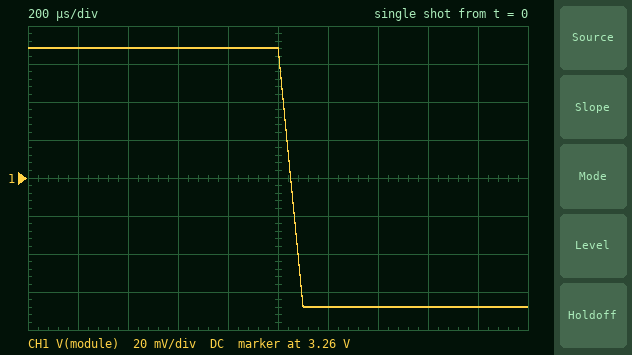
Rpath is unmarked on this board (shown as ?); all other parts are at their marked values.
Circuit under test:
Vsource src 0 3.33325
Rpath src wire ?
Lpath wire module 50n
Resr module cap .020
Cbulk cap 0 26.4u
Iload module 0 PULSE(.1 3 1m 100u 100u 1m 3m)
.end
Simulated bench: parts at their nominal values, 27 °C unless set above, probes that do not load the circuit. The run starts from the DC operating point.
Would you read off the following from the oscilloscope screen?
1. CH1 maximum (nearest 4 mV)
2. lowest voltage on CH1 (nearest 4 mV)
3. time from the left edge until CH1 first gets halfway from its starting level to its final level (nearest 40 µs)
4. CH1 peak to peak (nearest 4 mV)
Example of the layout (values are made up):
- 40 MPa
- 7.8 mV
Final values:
- 3.328 V
- 3.192 V
- 1.04 ms
- 136 mV
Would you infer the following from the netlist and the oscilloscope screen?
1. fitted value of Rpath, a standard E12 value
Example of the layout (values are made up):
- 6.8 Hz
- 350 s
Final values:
- 0.047 Ω
